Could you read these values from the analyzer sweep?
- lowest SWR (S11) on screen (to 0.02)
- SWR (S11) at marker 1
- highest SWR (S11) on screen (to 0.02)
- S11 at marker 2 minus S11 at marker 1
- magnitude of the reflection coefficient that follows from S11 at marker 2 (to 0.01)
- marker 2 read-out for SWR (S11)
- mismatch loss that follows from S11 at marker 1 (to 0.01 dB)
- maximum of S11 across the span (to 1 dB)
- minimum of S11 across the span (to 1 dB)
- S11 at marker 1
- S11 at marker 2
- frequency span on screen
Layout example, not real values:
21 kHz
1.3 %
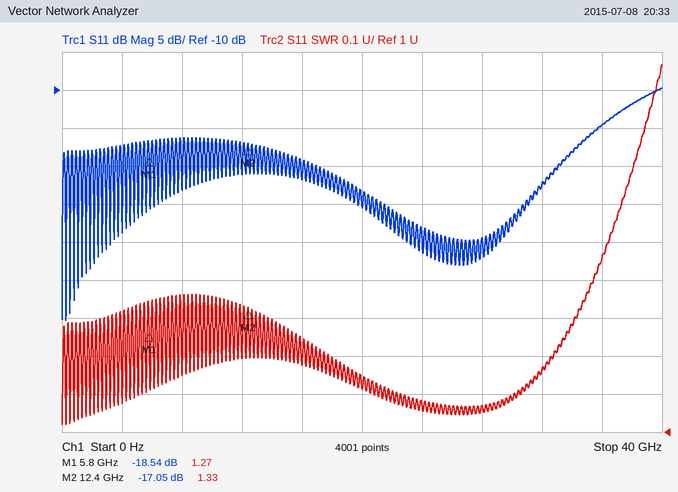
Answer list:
1.02
1.27
1.96
1.49 dB
0.14
1.33
0.06 dB
-10 dB
-40 dB
-18.54 dB
-17.05 dB
40 GHz
